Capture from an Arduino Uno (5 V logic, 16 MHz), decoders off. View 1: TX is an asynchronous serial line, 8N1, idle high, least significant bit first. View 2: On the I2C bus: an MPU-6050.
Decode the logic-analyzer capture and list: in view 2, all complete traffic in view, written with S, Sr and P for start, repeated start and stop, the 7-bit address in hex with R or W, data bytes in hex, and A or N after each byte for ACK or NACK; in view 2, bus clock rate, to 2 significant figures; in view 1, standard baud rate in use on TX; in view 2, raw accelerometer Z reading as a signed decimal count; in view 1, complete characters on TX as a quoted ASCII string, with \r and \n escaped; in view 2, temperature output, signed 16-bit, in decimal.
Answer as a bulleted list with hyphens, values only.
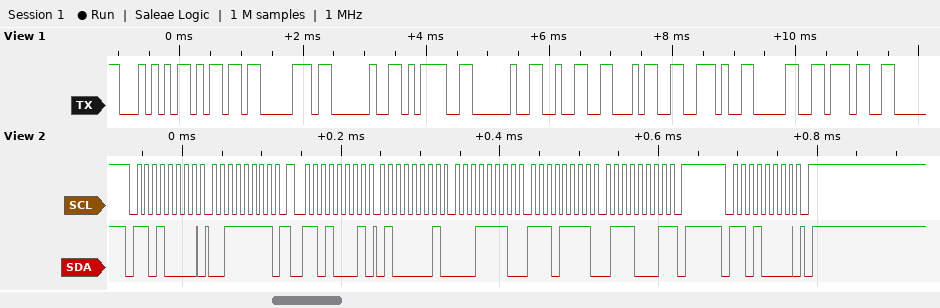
- S 68W A 3F A Sr 68R A 41 A 1E A EF A 71 N P S 68W A P
- 100 kHz
- 9600 baud
- 16670
- "Tmp = 24.07"
- -4239
